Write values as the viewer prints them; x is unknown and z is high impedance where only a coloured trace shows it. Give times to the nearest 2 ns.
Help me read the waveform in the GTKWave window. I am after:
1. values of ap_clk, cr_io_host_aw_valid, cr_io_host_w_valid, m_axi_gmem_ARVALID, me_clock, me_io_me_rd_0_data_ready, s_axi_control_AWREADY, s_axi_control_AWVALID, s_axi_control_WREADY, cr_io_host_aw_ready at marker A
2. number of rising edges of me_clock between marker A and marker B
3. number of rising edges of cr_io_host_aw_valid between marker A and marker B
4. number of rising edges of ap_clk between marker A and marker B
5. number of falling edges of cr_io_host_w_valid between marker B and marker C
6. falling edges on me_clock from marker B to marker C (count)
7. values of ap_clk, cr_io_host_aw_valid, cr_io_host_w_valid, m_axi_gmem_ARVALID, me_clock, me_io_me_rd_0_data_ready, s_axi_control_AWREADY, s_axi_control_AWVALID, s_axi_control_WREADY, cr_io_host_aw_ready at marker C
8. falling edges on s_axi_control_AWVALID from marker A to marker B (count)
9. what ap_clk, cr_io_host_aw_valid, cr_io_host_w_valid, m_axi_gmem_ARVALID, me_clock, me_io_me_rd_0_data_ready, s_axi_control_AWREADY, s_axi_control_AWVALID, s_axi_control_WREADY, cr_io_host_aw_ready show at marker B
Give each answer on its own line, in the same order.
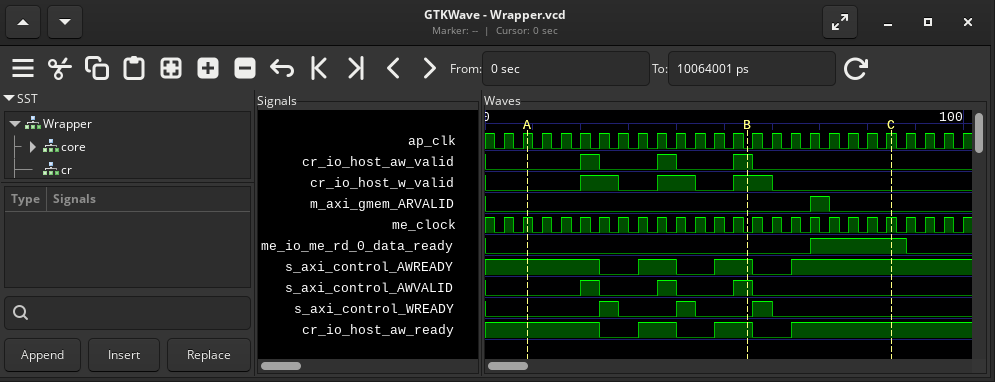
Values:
ap_clk=1, cr_io_host_aw_valid=0, cr_io_host_w_valid=0, m_axi_gmem_ARVALID=0, me_clock=1, me_io_me_rd_0_data_ready=0, s_axi_control_AWREADY=1, s_axi_control_AWVALID=0, s_axi_control_WREADY=0, cr_io_host_aw_ready=1
11
3
11
1
7
ap_clk=1, cr_io_host_aw_valid=0, cr_io_host_w_valid=0, m_axi_gmem_ARVALID=0, me_clock=1, me_io_me_rd_0_data_ready=1, s_axi_control_AWREADY=1, s_axi_control_AWVALID=0, s_axi_control_WREADY=0, cr_io_host_aw_ready=1
2
ap_clk=0, cr_io_host_aw_valid=1, cr_io_host_w_valid=1, m_axi_gmem_ARVALID=0, me_clock=0, me_io_me_rd_0_data_ready=0, s_axi_control_AWREADY=1, s_axi_control_AWVALID=1, s_axi_control_WREADY=0, cr_io_host_aw_ready=1
